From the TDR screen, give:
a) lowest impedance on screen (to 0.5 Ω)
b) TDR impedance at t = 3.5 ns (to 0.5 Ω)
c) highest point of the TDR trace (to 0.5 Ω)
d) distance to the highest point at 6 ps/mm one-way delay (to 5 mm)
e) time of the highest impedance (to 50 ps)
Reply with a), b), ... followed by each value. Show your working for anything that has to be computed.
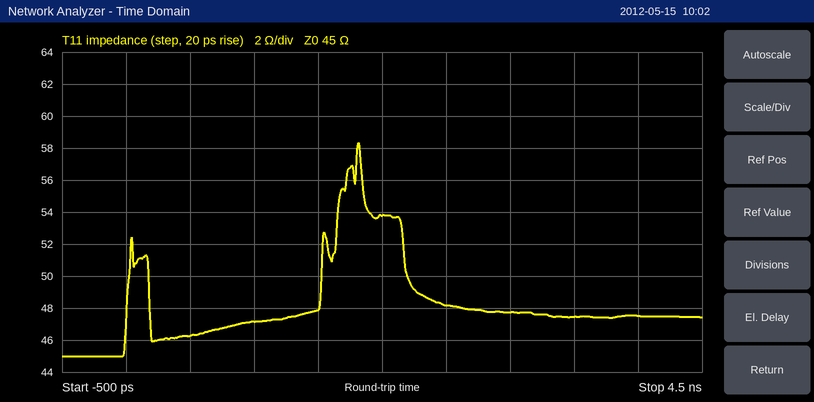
a) 45.0 Ω
b) 47.5 Ω
c) 58.5 Ω
d) 1.80 ns / 2 / 6 ps/mm ≈ 150 mm
e) 1.80 ns
